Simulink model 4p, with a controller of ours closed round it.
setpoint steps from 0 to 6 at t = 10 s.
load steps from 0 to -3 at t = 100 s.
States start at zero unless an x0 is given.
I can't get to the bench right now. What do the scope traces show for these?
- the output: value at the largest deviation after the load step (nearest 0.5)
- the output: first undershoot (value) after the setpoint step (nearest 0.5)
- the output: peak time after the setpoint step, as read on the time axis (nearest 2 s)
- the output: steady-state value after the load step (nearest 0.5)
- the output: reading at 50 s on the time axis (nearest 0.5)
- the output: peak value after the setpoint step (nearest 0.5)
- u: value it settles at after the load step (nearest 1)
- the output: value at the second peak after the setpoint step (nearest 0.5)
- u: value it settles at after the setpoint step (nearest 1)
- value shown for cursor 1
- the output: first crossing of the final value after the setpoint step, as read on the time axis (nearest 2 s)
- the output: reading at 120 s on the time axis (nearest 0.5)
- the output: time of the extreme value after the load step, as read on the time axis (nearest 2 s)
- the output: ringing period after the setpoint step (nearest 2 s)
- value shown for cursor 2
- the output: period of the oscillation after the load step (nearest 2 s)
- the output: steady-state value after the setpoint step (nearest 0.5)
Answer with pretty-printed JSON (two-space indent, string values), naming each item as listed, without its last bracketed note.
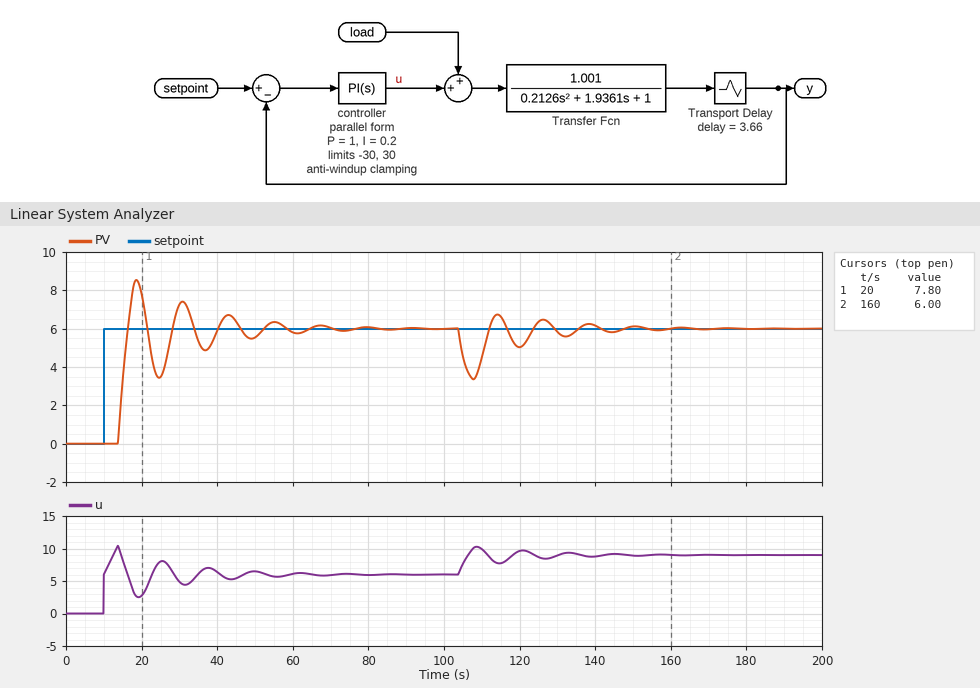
{
  "the output: value at the largest deviation after the load step": "3.5",
  "the output: first undershoot (value) after the setpoint step": "3.5",
  "the output: peak time after the setpoint step, as read on the time axis": "18 s",
  "the output: steady-state value after the load step": "6.0",
  "the output: reading at 50 s on the time axis": "5.5",
  "the output: peak value after the setpoint step": "8.5",
  "u: value it settles at after the load step": "9",
  "the output: value at the second peak after the setpoint step": "7.5",
  "u: value it settles at after the setpoint step": "6",
  "value shown for cursor 1": "7.80",
  "the output: first crossing of the final value after the setpoint step, as read on the time axis": "16 s",
  "the output: reading at 120 s on the time axis": "5.0",
  "the output: time of the extreme value after the load step, as read on the time axis": "108 s",
  "the output: ringing period after the setpoint step": "12 s",
  "value shown for cursor 2": "6.00",
  "the output: period of the oscillation after the load step": "12 s",
  "the output: steady-state value after the setpoint step": "6.0"
}
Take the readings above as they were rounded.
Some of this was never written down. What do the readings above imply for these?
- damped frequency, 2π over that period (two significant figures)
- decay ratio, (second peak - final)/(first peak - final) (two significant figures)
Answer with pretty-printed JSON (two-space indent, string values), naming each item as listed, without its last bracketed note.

{
  "damped frequency, 2π over that period": "0.52 rad/s",
  "decay ratio, (second peak - final)/(first peak - final)": "0.60"
}
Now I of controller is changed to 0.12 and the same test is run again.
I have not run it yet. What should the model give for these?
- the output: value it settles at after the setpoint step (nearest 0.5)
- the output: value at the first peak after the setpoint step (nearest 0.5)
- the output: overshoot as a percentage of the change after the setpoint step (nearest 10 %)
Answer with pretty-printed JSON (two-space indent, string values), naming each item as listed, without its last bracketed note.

{
  "the output: value it settles at after the setpoint step": "6.0",
  "the output: value at the first peak after the setpoint step": "7.0",
  "the output: overshoot as a percentage of the change after the setpoint step": "20 %"
}
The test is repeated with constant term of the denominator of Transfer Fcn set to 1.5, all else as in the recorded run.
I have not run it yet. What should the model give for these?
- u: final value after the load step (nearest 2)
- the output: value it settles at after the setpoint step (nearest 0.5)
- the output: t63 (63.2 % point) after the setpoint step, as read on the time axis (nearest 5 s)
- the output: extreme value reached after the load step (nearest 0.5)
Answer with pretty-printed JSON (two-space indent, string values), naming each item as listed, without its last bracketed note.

{
  "u: final value after the load step": "12",
  "the output: value it settles at after the setpoint step": "6.0",
  "the output: t63 (63.2 % point) after the setpoint step, as read on the time axis": "15 s",
  "the output: extreme value reached after the load step": "4.0"
}
